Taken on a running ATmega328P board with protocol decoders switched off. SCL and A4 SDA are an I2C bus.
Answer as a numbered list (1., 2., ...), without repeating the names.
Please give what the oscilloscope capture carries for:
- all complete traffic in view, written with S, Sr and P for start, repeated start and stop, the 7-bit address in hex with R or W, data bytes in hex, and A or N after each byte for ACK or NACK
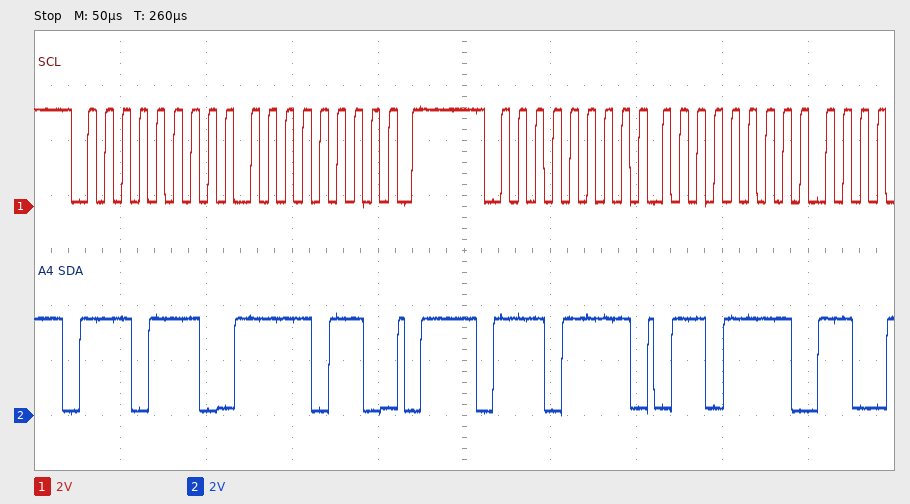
1. S 77W A F6 A P S 77R A 6F A
